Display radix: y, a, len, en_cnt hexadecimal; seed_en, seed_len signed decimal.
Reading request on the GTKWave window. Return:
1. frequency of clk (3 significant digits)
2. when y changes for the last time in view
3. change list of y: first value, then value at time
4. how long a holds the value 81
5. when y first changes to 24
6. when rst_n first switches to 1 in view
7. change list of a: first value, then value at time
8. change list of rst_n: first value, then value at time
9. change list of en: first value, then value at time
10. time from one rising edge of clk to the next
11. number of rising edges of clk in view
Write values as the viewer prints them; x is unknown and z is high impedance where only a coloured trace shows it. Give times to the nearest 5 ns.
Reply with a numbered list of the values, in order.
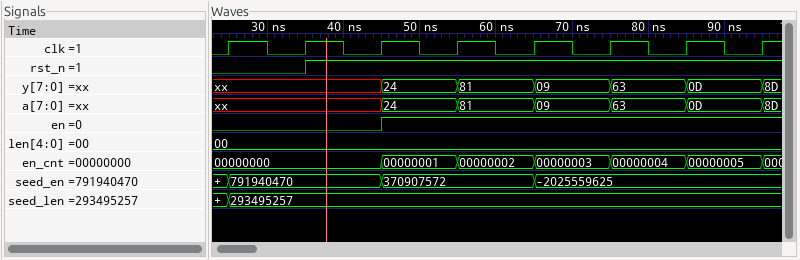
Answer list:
1. 100 MHz
2. 95 ns
3. xx, 24 at 45 ns, 81 at 55 ns, 09 at 65 ns, 63 at 75 ns, 0D at 85 ns, 8D at 95 ns
4. 10 ns
5. 45 ns
6. 35 ns
7. xx, 24 at 45 ns, 81 at 55 ns, 09 at 65 ns, 63 at 75 ns, 0D at 85 ns, 8D at 95 ns
8. 0, 1 at 35 ns
9. 0, 1 at 45 ns
10. 10 ns
11. 8
